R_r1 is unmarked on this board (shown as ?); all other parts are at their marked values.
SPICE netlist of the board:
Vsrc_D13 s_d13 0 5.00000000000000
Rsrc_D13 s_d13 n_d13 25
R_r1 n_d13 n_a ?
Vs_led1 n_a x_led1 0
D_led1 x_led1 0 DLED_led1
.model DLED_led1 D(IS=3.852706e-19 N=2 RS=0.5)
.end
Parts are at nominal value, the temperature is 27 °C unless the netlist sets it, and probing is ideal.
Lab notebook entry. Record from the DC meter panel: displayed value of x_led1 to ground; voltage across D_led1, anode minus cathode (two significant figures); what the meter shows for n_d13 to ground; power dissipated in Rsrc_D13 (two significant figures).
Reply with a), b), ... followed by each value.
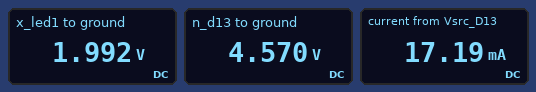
a) 1.992 V
b) 2.0 V
c) 4.570 V
d) 7.4 mW
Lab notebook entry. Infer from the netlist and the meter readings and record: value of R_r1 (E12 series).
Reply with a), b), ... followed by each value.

a) 150 Ω
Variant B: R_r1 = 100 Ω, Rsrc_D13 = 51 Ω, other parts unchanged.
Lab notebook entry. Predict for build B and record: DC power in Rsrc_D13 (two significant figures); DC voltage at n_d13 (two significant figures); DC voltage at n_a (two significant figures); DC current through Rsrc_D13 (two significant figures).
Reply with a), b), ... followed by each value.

a) 20 mW
b) 4.0 V
c) 2.0 V
d) 20 mA
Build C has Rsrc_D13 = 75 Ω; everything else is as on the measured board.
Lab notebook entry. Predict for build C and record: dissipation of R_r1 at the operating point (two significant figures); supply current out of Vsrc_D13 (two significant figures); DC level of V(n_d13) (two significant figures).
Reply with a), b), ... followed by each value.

a) 27 mW
b) 13 mA
c) 4.0 V
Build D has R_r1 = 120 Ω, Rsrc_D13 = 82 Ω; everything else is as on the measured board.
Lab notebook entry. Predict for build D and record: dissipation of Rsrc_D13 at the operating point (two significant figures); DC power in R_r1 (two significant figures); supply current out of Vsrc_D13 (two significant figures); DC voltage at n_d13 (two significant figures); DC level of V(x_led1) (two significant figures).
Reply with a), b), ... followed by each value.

a) 18 mW
b) 27 mW
c) 15 mA
d) 3.8 V
e) 2.0 V
